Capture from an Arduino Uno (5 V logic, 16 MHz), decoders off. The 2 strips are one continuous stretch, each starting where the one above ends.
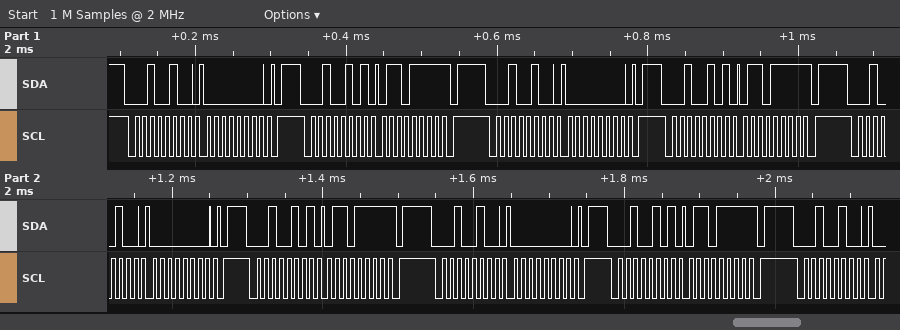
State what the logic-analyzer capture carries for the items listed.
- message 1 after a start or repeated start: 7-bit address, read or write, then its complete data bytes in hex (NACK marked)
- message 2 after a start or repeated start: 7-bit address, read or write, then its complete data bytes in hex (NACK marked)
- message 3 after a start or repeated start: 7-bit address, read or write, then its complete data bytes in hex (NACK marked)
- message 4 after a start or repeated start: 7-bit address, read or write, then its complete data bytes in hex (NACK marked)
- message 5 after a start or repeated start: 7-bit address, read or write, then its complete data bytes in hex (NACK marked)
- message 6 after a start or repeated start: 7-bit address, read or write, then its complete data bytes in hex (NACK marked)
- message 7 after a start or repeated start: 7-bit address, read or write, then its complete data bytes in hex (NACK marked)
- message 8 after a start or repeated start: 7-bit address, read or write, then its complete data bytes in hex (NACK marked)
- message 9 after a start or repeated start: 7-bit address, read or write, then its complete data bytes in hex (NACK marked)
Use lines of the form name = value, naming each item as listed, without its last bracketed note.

message 1 after a start or repeated start: 7-bit address, read or write, then its complete data bytes in hex = 0x12 write: 00
message 2 after a start or repeated start: 7-bit address, read or write, then its complete data bytes in hex = 0x12 read: 6F NACK
message 3 after a start or repeated start: 7-bit address, read or write, then its complete data bytes in hex = 0x12 write: 00
message 4 after a start or repeated start: 7-bit address, read or write, then its complete data bytes in hex = 0x12 read: 6F NACK
message 5 after a start or repeated start: 7-bit address, read or write, then its complete data bytes in hex = 0x12 write: 00
message 6 after a start or repeated start: 7-bit address, read or write, then its complete data bytes in hex = 0x12 read: 6F NACK
message 7 after a start or repeated start: 7-bit address, read or write, then its complete data bytes in hex = 0x12 write: 00
message 8 after a start or repeated start: 7-bit address, read or write, then its complete data bytes in hex = 0x12 read: 6F NACK
message 9 after a start or repeated start: 7-bit address, read or write, then its complete data bytes in hex = 0x12 write
